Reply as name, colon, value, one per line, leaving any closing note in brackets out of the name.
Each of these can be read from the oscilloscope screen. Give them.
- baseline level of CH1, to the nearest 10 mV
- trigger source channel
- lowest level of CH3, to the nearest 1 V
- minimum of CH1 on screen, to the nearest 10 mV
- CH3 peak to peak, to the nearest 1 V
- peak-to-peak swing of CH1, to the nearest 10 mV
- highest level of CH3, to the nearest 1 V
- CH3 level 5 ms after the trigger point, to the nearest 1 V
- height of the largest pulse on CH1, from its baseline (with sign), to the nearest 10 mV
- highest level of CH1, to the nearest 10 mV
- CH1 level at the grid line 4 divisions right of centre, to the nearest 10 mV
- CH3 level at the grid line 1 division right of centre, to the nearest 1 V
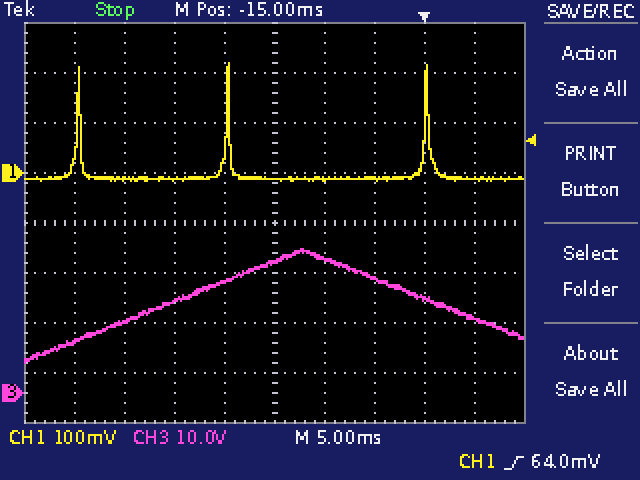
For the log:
baseline level of CH1, to the nearest 10 mV: -10 mV
trigger source channel: CH1
lowest level of CH3, to the nearest 1 V: 6 V
minimum of CH1 on screen, to the nearest 10 mV: -20 mV
CH3 peak to peak, to the nearest 1 V: 23 V
peak-to-peak swing of CH1, to the nearest 10 mV: 240 mV
highest level of CH3, to the nearest 1 V: 29 V
CH3 level 5 ms after the trigger point, to the nearest 1 V: 15 V
height of the largest pulse on CH1, from its baseline (with sign), to the nearest 10 mV: +230 mV
highest level of CH1, to the nearest 10 mV: 220 mV
CH1 level at the grid line 4 divisions right of centre, to the nearest 10 mV: -10 mV
CH3 level at the grid line 1 division right of centre, to the nearest 1 V: 27 V
